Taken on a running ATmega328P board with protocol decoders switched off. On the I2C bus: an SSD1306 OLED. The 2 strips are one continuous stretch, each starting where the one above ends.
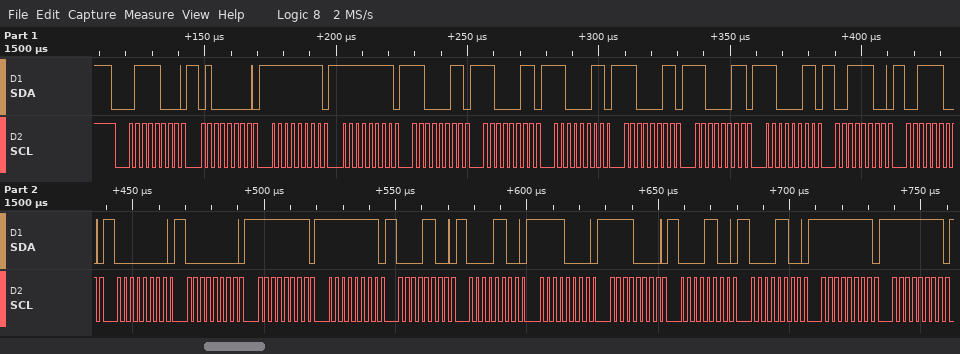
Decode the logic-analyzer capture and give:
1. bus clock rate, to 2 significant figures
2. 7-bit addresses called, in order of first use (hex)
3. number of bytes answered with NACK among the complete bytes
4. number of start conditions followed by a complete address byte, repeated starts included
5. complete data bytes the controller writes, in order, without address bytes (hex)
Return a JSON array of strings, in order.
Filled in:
["400 kHz", "0x3C", "0", "1", "40 FF FF C3 C3 C3 C3 C3 C3 3C 3C 00 00 FF FF 0C 0C F0 F0 0C 0C FF FF"]
